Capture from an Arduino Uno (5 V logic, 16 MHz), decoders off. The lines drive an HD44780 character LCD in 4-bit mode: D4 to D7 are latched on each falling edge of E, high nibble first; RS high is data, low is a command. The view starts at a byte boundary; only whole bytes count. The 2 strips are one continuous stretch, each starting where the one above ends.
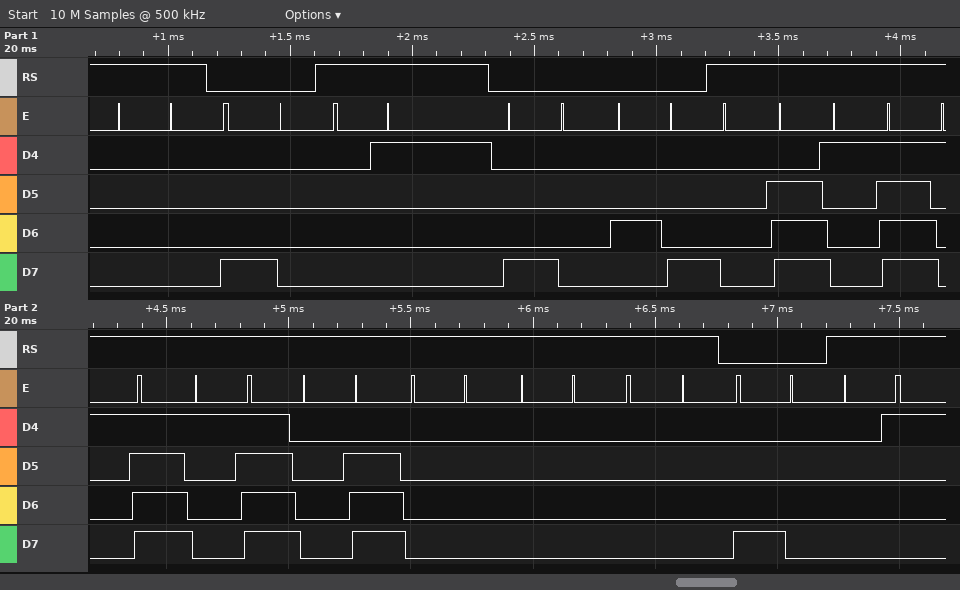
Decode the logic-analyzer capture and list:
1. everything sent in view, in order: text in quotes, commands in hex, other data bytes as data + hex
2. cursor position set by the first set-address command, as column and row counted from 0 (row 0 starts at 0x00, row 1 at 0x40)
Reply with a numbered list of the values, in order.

1. data 00 0x80 data 01 0x80 0x48 data 0E 1F 1F 1F 0E 00 00 00 0x80 data 01
2. column 0, row 0
